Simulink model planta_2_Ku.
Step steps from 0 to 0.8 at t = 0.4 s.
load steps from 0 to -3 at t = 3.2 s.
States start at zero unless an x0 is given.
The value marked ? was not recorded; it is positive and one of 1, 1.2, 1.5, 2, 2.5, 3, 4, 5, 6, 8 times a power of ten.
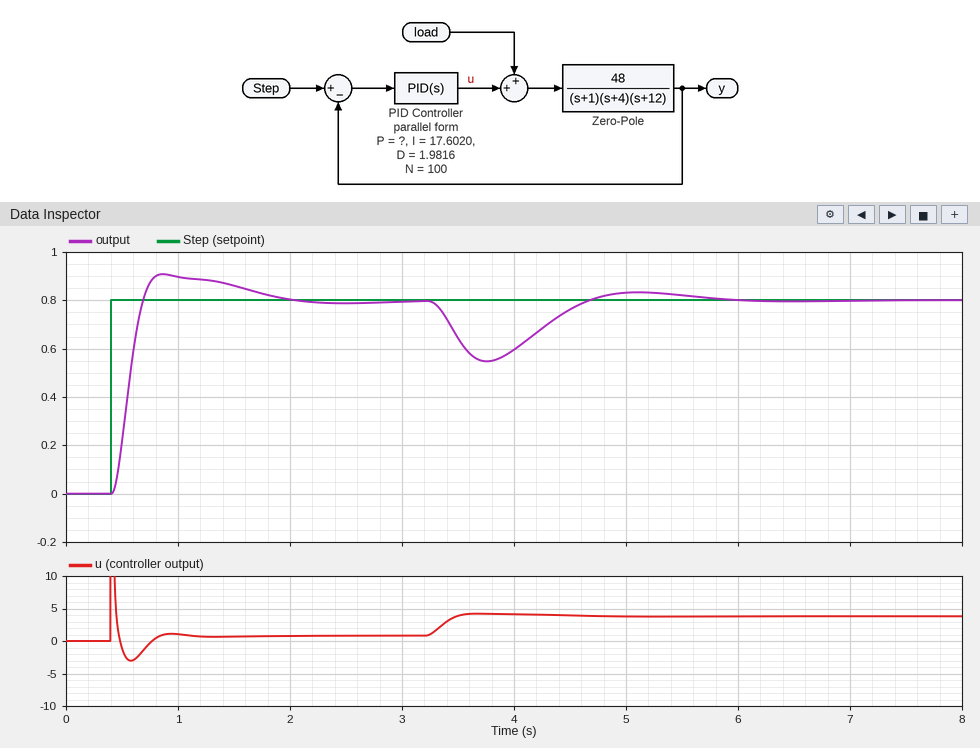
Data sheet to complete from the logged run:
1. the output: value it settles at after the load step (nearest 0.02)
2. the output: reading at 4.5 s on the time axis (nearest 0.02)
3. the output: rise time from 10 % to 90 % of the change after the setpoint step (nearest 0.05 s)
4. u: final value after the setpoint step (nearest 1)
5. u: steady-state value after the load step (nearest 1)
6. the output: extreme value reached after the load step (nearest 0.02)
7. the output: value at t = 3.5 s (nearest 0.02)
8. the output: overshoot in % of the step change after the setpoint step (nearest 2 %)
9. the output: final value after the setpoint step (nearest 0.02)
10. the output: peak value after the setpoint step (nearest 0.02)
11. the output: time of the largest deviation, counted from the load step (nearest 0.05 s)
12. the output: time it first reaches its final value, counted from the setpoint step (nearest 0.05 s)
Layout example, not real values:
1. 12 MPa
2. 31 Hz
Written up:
1. 0.80
2. 0.76
3. 0.20 s
4. 1
5. 4
6. 0.54
7. 0.64
8. 14 %
9. 0.80
10. 0.90
11. 0.55 s
12. 0.30 s
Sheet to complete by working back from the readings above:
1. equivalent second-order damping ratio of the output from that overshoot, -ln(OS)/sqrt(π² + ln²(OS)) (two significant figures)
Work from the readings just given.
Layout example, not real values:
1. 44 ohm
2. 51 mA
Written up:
1. 0.53
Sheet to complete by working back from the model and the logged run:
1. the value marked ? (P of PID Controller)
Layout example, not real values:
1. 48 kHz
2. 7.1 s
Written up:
1. 8
